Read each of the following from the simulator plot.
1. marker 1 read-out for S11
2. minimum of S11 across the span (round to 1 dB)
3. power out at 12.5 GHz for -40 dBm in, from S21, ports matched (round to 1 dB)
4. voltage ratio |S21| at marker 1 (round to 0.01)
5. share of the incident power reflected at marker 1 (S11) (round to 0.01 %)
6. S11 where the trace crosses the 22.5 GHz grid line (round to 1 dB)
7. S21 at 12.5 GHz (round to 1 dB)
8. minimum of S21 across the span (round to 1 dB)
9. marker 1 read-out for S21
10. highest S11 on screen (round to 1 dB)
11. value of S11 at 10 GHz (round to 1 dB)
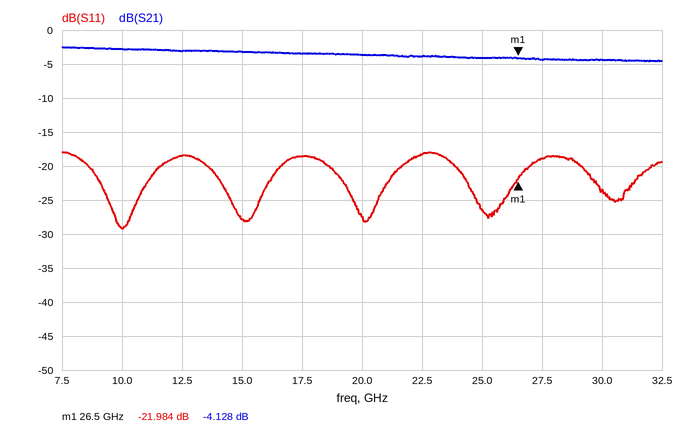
-21.984 dB
-29 dB
-43 dBm
0.62
0.63 %
-18 dB
-3 dB
-5 dB
-4.128 dB
-18 dB
-29 dB
